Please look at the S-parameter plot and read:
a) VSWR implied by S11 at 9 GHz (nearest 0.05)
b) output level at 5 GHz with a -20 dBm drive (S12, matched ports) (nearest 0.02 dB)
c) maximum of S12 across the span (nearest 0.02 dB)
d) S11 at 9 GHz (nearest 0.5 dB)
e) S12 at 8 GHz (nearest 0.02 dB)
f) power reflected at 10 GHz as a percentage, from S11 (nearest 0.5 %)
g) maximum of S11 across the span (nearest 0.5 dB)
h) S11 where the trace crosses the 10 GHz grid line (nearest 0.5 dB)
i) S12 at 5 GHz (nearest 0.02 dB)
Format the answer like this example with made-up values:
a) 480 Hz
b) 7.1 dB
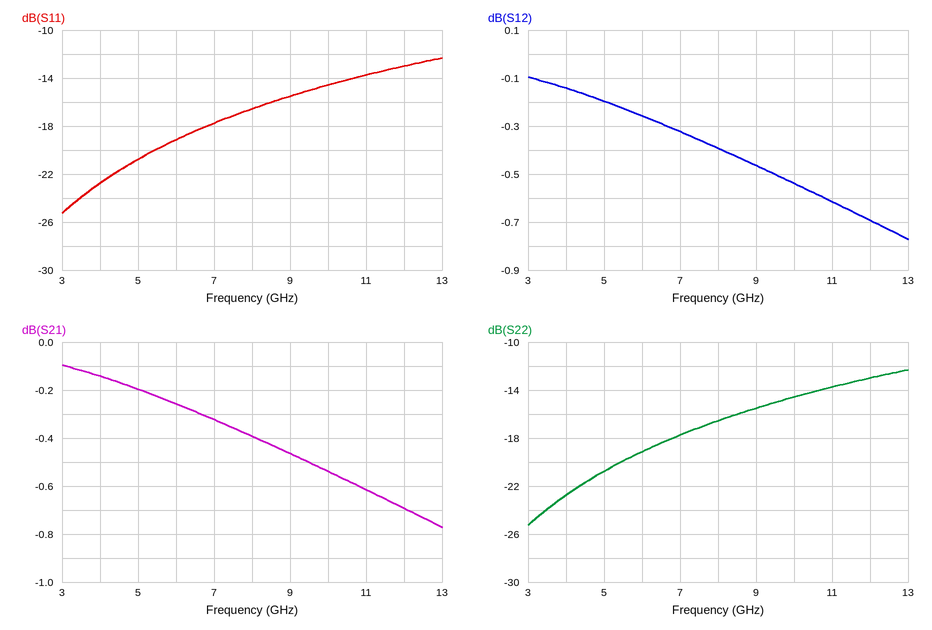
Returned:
a) 1.40
b) -20.20 dBm
c) -0.10 dB
d) -15.5 dB
e) -0.40 dB
f) 3.5 %
g) -12.5 dB
h) -14.5 dB
i) -0.20 dB
